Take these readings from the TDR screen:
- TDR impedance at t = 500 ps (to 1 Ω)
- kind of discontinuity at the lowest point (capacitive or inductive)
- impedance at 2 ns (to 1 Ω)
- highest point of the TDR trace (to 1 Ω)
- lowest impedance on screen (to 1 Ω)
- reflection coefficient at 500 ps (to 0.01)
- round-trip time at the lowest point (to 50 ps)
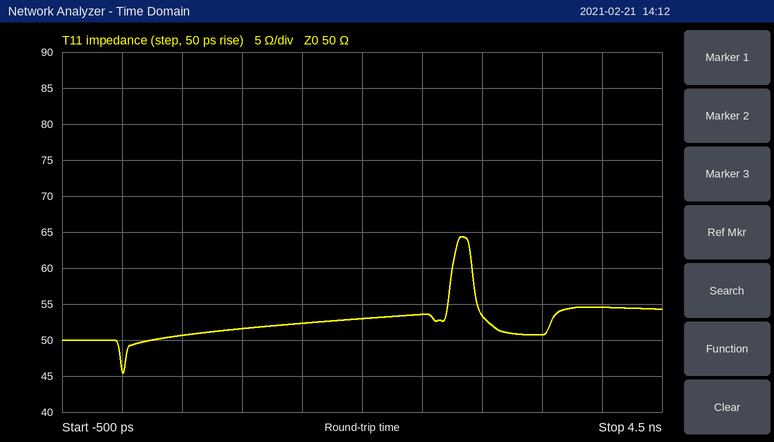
51 Ω
capacitive
53 Ω
64 Ω
45 Ω
+0.01
0 ps
